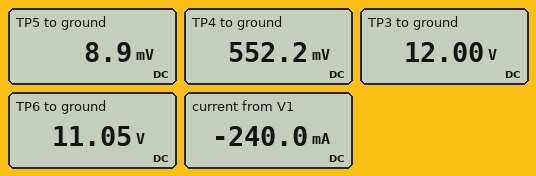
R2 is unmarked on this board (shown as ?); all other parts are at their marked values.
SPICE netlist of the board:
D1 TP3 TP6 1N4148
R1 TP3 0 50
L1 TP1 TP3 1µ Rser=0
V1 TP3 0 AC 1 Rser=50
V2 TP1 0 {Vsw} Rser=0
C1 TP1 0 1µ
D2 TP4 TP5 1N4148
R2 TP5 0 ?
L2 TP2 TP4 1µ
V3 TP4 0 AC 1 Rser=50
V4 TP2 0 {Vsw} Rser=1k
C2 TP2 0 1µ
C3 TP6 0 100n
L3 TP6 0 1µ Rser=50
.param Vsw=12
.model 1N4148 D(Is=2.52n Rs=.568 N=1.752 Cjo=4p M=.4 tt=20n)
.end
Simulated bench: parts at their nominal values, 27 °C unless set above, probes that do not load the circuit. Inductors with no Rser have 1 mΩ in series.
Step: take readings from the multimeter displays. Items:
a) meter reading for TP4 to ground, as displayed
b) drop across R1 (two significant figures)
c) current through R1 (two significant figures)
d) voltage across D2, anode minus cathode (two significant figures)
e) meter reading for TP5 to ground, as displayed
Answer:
552.2 mV
12 V
240 mA
540 mV
8.9 mV
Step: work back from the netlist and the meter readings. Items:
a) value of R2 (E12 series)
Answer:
22 Ω
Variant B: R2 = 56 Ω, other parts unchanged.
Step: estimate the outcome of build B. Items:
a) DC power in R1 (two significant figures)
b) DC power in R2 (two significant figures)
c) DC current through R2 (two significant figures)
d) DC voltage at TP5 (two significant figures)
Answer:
2.9 W
6.6 µW
340 µA
19 mV
